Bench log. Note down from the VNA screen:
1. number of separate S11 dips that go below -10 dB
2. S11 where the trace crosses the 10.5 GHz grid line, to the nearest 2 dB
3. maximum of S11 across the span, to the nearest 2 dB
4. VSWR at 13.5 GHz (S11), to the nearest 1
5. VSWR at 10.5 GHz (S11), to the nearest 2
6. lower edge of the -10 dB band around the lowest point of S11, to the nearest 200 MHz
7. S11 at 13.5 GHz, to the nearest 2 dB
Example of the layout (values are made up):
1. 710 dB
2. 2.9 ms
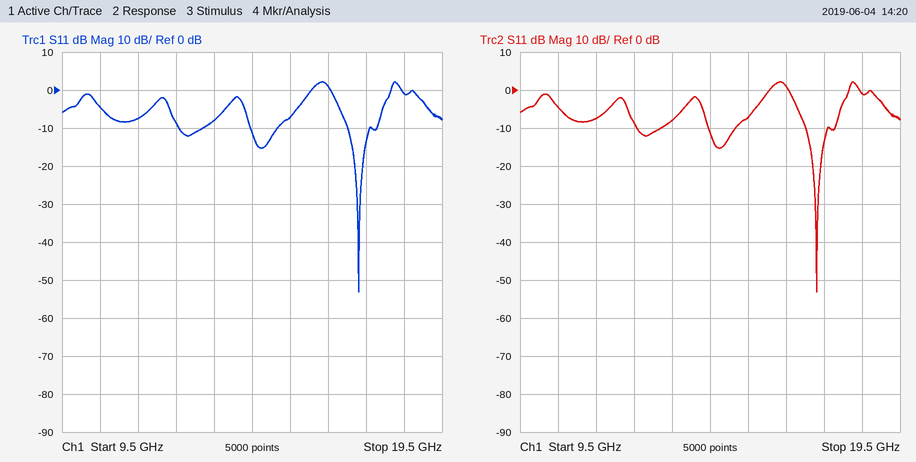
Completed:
1. 3
2. -4 dB
3. 2 dB
4. 2
5. 4
6. 17.0 GHz
7. -8 dB
